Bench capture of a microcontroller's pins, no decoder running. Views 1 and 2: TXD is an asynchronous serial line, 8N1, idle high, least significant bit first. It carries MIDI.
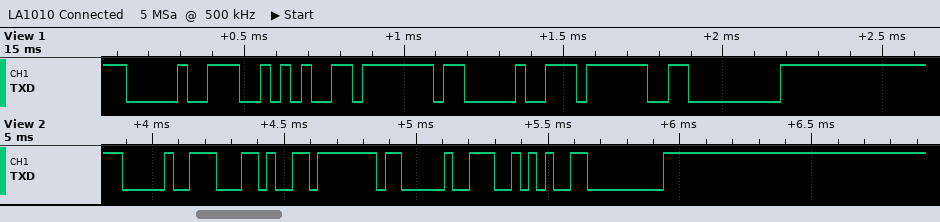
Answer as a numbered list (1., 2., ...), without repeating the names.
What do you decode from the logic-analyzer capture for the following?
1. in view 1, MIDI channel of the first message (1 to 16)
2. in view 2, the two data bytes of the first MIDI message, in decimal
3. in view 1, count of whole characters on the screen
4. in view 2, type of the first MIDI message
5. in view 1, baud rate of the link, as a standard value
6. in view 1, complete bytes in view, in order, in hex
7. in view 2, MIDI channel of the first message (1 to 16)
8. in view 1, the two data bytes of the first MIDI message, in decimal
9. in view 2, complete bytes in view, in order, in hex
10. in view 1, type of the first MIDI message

1. 1
2. 44, 127
3. 6
4. Note On
5. 31250 baud
6. 90 2A 7F 90 3F 00
7. 1
8. 42, 127
9. 90 2C 7F 90 2A 00
10. Note On
